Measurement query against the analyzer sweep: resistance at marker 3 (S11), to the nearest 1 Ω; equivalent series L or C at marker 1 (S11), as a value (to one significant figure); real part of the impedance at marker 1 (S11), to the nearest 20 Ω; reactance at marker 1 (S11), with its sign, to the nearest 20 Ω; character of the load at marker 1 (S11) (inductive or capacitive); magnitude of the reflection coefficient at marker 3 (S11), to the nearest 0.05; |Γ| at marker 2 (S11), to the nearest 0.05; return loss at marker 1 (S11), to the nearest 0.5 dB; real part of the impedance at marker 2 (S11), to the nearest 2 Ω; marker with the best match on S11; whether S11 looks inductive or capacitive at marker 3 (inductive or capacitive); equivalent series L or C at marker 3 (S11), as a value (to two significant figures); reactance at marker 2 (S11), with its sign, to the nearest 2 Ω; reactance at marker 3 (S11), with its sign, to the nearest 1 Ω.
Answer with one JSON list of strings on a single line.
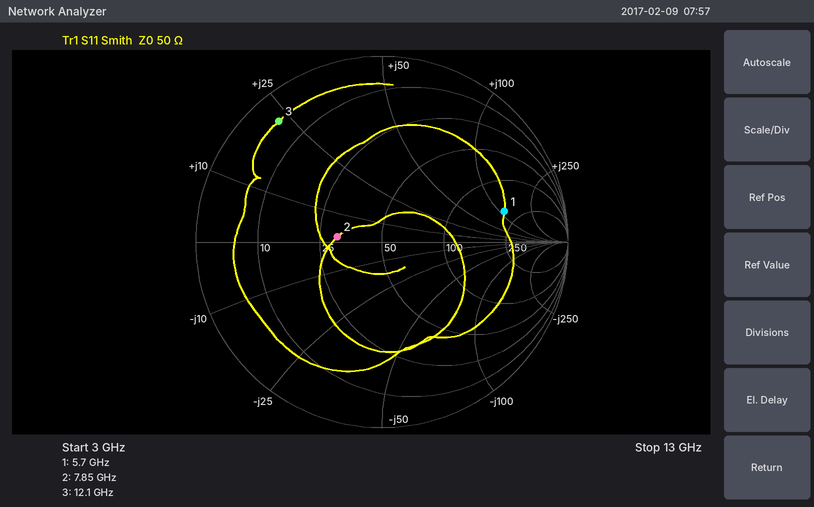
["5 Ω", "3 nH", "180 Ω", "+120 Ω", "inductive", "0.85", "0.25", "3.5 dB", "30 Ω", "marker 2", "inductive", "300 pH", "+2 Ω", "+23 Ω"]
